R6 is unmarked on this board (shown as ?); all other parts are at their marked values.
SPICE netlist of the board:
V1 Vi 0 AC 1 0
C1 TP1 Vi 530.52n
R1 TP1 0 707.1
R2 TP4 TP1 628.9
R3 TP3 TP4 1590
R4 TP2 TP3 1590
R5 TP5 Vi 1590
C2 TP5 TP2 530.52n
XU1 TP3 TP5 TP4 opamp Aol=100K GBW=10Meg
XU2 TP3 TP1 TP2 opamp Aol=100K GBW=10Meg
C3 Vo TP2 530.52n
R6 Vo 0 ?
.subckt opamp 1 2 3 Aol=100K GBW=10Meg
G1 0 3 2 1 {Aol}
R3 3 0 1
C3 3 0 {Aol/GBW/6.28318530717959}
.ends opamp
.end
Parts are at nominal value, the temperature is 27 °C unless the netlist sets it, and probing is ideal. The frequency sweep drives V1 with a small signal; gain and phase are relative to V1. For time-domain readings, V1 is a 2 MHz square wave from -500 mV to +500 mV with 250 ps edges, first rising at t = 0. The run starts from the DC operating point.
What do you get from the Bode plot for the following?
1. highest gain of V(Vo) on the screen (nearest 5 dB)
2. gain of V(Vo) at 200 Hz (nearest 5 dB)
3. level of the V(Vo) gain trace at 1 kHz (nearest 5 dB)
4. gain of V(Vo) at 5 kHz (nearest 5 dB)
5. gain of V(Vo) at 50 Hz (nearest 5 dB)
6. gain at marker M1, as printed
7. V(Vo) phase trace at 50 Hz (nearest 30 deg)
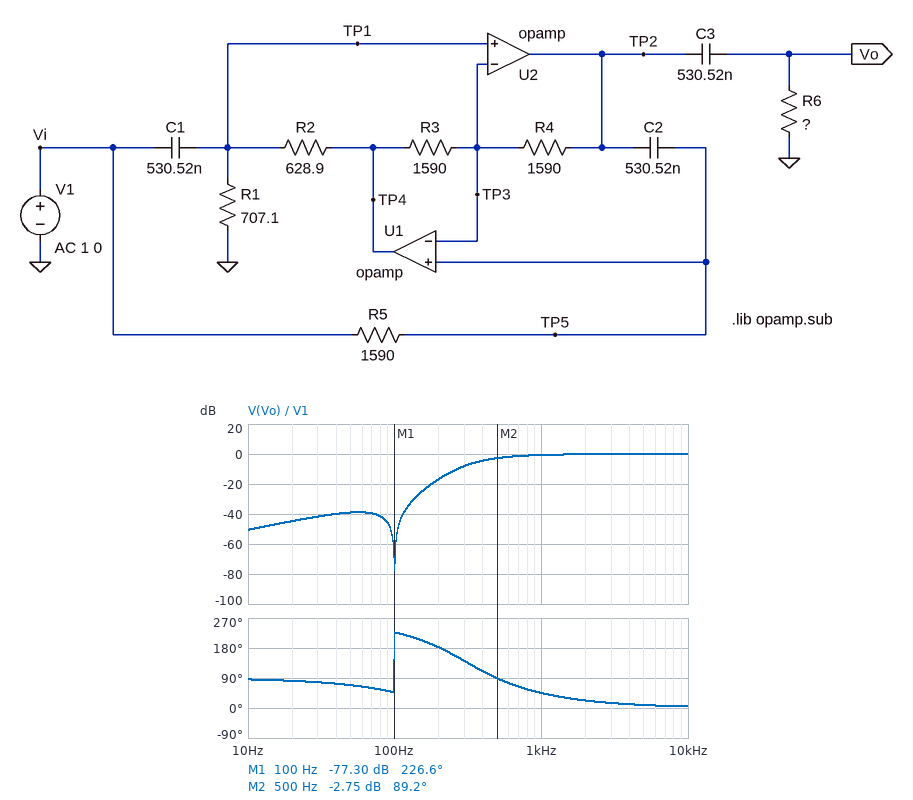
0 dB
-15 dB
0 dB
0 dB
-40 dB
-77.30 dB
60 deg
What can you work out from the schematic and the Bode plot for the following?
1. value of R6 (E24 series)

820 Ω
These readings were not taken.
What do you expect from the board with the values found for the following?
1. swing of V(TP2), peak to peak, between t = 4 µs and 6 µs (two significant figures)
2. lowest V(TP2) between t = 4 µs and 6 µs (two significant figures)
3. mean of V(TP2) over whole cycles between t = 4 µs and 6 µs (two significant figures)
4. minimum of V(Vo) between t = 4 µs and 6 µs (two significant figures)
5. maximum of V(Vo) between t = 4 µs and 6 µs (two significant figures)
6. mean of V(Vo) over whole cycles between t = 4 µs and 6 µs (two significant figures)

1.4 V
-270 mV
440 mV
-220 mV
1.2 V
490 mV
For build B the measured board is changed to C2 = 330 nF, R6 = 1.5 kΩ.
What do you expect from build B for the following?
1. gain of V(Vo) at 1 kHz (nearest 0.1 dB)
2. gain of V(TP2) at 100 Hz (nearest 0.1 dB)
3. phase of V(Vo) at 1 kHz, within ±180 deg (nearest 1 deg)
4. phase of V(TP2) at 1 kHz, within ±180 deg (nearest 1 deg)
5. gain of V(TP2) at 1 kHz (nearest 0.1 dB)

0.1 dB
-27.4 dB
38 deg
26 deg
0.3 dB
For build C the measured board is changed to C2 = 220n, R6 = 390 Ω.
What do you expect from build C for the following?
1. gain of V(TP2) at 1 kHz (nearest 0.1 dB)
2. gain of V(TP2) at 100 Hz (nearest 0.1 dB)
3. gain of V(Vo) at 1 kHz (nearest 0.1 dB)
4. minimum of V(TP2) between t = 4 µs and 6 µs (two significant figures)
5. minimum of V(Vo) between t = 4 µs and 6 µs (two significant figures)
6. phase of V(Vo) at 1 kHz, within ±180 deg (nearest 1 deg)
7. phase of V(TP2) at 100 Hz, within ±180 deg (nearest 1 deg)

0.8 dB
-23.6 dB
-1.2 dB
-270 mV
-230 mV
66 deg
-12 deg
